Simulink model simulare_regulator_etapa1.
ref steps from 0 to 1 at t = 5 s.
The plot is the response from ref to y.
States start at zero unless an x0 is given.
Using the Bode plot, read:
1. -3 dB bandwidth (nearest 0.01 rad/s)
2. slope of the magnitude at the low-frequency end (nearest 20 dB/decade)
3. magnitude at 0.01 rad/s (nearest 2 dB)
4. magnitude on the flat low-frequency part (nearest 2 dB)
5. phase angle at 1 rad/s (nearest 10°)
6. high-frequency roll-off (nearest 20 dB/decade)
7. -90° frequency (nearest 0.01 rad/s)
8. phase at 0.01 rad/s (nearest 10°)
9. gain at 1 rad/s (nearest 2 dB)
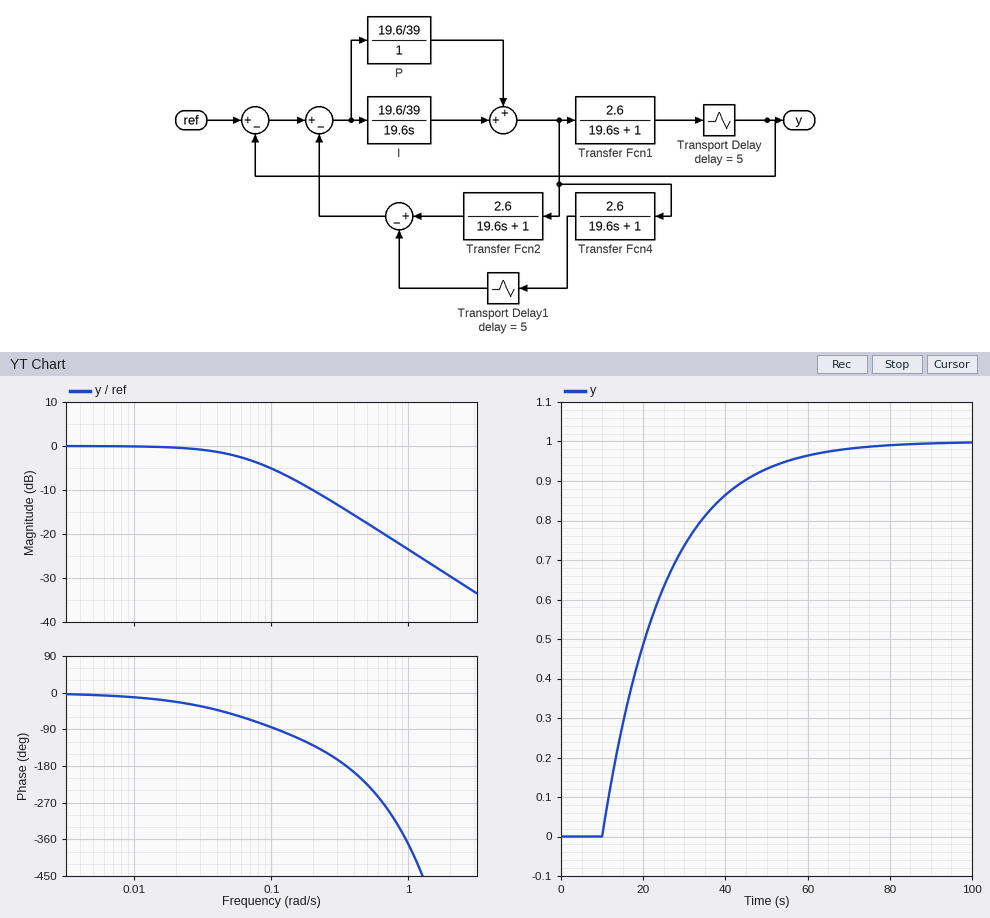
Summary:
0.07 rad/s
0 dB/decade
0 dB
0 dB
-370°
-20 dB/decade
0.11 rad/s
-10°
-24 dB
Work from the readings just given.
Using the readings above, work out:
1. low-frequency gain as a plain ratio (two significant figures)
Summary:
1.0
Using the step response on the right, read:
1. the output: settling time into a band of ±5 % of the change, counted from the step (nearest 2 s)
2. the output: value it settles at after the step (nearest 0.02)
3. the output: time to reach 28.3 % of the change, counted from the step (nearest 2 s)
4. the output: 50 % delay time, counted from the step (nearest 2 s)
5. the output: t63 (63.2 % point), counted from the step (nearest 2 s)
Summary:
50 s
1.00
10 s
16 s
20 s
